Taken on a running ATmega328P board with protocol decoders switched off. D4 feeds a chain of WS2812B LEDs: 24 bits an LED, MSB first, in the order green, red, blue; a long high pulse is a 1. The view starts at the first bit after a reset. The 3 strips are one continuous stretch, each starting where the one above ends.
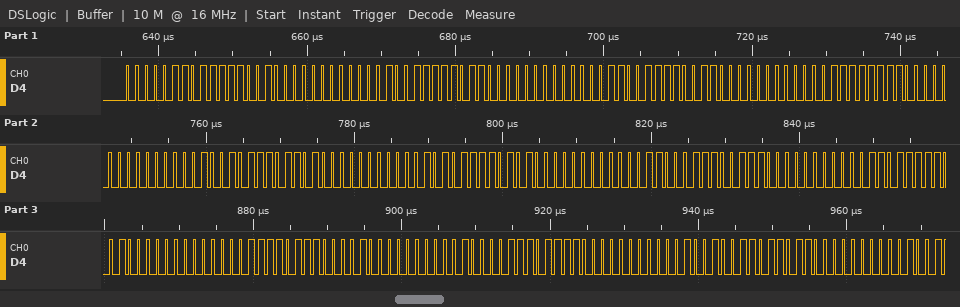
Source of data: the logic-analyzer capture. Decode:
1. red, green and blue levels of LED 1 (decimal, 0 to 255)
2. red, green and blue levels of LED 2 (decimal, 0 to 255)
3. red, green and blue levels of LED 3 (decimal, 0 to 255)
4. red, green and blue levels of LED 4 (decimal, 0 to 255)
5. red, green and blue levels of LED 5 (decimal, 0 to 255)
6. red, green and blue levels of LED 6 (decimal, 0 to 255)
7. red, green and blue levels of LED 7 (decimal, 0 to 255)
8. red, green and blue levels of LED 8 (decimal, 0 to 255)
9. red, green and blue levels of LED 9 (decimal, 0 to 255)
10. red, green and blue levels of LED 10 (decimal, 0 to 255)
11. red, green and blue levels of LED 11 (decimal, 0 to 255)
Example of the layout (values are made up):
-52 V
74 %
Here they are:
249, 6, 0
246, 9, 0
243, 12, 0
240, 15, 0
237, 18, 0
234, 21, 0
231, 24, 0
228, 27, 0
225, 30, 0
222, 33, 0
219, 36, 0
